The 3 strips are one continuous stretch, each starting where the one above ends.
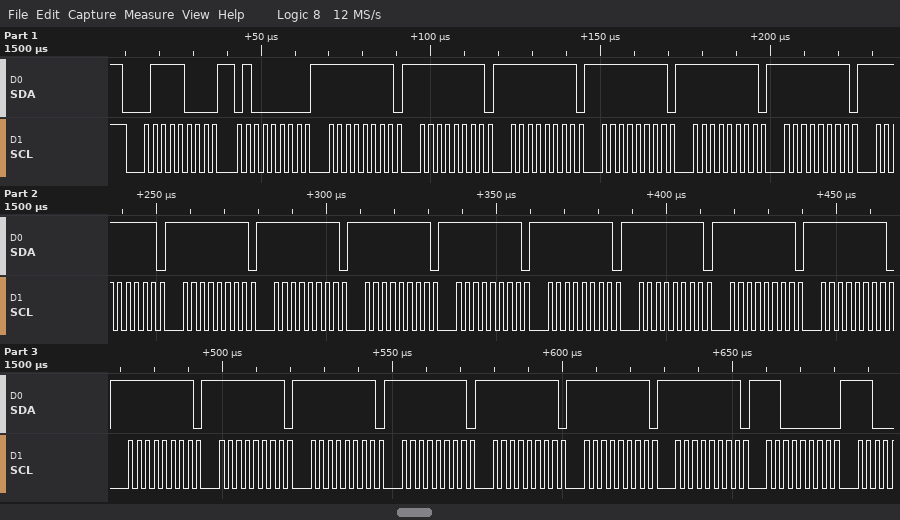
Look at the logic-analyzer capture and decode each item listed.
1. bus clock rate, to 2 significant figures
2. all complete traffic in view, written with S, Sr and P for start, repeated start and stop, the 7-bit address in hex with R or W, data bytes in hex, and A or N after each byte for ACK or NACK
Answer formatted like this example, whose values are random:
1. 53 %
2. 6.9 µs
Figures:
1. 400 kHz
2. S 3CW A 40 A FF A FF A FF A FF A FF A FF A FF A FF A FF A FF A FF A FF A FF A FF A FF A FF A FF A FF A FF A FF A FF A FF A C0 A
